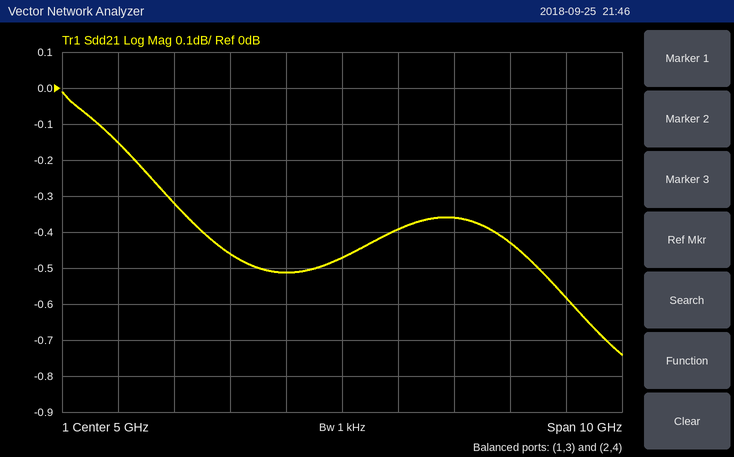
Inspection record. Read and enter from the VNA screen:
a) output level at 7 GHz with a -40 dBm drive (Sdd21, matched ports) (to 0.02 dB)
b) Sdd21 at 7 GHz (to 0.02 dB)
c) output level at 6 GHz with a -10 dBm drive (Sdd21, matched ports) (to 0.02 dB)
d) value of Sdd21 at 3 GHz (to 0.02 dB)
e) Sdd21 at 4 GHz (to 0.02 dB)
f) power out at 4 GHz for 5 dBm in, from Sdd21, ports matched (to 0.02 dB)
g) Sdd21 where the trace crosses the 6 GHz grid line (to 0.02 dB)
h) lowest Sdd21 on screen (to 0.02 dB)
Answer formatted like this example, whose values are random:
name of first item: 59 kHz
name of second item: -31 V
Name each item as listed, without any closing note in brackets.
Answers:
output level at 7 GHz with a -40 dBm drive (Sdd21, matched ports): -40.36 dBm
Sdd21 at 7 GHz: -0.36 dB
output level at 6 GHz with a -10 dBm drive (Sdd21, matched ports): -10.40 dBm
value of Sdd21 at 3 GHz: -0.46 dB
Sdd21 at 4 GHz: -0.52 dB
power out at 4 GHz for 5 dBm in, from Sdd21, ports matched: 4.48 dBm
Sdd21 where the trace crosses the 6 GHz grid line: -0.40 dB
lowest Sdd21 on screen: -0.74 dB
